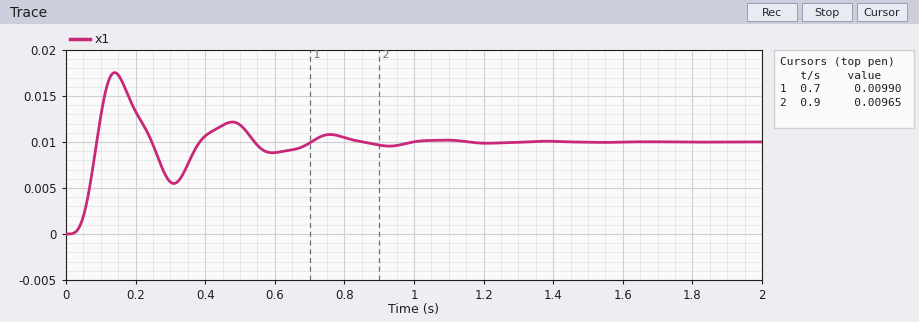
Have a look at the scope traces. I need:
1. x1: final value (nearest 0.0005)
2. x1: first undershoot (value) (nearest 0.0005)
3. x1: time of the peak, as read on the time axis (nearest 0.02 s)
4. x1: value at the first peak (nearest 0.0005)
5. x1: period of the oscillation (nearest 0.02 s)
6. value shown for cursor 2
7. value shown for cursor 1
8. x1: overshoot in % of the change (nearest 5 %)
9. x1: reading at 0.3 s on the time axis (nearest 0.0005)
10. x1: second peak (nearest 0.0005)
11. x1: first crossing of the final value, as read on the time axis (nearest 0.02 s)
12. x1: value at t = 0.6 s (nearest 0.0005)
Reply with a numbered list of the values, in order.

1. 0.0100
2. 0.0055
3. 0.14 s
4. 0.0175
5. 0.34 s
6. 0.00965
7. 0.00990
8. 75 %
9. 0.0055
10. 0.0120
11. 0.08 s
12. 0.0090
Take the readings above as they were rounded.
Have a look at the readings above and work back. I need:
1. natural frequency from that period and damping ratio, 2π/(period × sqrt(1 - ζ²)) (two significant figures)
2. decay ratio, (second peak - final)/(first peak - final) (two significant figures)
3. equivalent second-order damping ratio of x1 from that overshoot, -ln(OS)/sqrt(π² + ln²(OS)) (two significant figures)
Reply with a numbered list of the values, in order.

1. 19 rad/s
2. 0.27
3. 0.091
